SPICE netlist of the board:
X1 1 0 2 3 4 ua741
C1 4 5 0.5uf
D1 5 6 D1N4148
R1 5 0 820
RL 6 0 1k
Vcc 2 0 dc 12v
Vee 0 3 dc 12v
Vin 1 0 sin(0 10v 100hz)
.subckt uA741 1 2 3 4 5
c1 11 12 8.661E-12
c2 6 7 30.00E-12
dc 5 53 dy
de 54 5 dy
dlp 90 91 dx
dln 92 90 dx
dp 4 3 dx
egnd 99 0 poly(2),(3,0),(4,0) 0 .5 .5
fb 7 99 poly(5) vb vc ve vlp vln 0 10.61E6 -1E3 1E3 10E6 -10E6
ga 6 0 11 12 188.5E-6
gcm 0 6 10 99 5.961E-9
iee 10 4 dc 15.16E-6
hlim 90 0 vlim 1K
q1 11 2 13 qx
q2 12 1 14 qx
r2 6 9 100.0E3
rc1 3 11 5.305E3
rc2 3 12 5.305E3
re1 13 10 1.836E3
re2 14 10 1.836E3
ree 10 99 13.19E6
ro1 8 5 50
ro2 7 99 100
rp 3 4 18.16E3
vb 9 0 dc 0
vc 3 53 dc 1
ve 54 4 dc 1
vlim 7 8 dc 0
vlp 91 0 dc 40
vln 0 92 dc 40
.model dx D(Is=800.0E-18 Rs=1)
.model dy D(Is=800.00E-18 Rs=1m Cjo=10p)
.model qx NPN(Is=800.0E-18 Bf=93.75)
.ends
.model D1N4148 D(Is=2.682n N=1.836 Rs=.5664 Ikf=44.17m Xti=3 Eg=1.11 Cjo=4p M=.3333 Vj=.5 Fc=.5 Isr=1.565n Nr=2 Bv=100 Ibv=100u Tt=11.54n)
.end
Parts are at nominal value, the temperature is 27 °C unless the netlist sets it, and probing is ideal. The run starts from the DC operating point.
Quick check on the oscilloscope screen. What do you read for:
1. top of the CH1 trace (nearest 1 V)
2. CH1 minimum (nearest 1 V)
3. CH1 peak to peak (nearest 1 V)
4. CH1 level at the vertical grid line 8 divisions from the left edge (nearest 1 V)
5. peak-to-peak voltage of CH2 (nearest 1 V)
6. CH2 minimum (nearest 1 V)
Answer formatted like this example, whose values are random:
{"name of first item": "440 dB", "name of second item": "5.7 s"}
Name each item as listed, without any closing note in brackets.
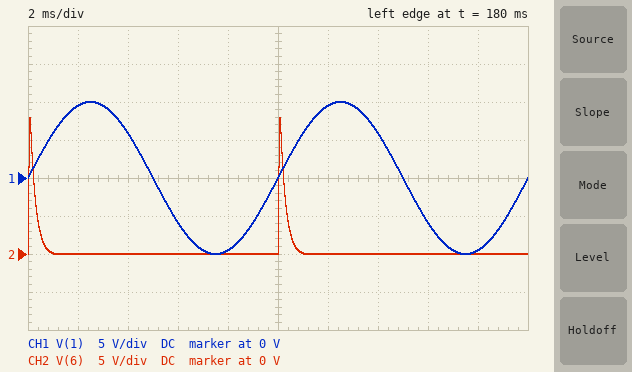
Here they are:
{"top of the CH1 trace": "10 V", "CH1 minimum": "-10 V", "CH1 peak to peak": "20 V", "CH1 level at the vertical grid line 8 divisions from the left edge": "-6 V", "peak-to-peak voltage of CH2": "18 V", "CH2 minimum": "0 V"}
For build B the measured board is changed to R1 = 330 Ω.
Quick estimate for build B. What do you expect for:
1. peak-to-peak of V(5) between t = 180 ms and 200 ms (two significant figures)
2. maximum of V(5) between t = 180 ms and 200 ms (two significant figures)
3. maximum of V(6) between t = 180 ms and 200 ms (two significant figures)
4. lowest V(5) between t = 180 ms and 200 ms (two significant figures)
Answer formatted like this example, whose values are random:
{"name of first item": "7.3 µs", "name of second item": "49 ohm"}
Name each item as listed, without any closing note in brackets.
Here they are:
{"peak-to-peak of V(5) between t = 180 ms and 200 ms": "24 V", "maximum of V(5) between t = 180 ms and 200 ms": "10 V", "maximum of V(6) between t = 180 ms and 200 ms": "9.5 V", "lowest V(5) between t = 180 ms and 200 ms": "-13 V"}
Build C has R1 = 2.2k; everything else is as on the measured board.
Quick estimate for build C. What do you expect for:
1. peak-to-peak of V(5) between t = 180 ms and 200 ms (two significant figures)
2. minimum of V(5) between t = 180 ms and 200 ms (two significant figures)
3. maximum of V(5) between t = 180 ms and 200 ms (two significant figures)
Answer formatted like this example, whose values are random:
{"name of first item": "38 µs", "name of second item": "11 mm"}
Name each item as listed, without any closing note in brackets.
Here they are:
{"peak-to-peak of V(5) between t = 180 ms and 200 ms": "45 V", "minimum of V(5) between t = 180 ms and 200 ms": "-23 V", "maximum of V(5) between t = 180 ms and 200 ms": "22 V"}
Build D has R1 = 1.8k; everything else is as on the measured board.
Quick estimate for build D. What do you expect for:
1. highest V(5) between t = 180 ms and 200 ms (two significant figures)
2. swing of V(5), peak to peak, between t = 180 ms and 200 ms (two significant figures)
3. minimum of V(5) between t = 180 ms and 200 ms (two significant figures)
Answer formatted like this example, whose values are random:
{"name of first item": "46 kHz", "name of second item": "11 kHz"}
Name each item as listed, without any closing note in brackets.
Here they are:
{"highest V(5) between t = 180 ms and 200 ms": "22 V", "swing of V(5), peak to peak, between t = 180 ms and 200 ms": "45 V", "minimum of V(5) between t = 180 ms and 200 ms": "-23 V"}
